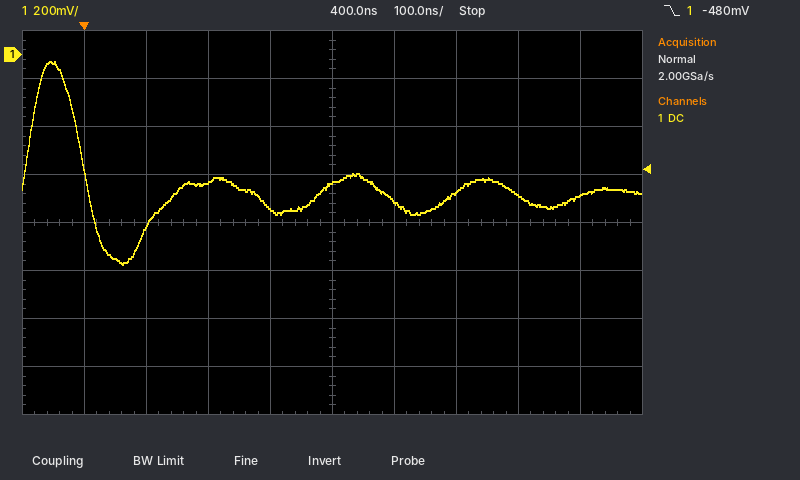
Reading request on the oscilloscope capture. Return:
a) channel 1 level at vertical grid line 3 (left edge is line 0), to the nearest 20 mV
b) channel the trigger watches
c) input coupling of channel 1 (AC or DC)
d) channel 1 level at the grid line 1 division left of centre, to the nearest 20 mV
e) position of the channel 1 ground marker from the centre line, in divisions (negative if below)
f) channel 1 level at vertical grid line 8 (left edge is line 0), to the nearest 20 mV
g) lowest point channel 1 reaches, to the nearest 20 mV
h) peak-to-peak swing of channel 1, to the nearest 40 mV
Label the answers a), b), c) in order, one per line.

a) -540 mV
b) channel 1
c) DC
d) -640 mV
e) +3.5 div
f) -580 mV
g) -880 mV
h) 840 mV
